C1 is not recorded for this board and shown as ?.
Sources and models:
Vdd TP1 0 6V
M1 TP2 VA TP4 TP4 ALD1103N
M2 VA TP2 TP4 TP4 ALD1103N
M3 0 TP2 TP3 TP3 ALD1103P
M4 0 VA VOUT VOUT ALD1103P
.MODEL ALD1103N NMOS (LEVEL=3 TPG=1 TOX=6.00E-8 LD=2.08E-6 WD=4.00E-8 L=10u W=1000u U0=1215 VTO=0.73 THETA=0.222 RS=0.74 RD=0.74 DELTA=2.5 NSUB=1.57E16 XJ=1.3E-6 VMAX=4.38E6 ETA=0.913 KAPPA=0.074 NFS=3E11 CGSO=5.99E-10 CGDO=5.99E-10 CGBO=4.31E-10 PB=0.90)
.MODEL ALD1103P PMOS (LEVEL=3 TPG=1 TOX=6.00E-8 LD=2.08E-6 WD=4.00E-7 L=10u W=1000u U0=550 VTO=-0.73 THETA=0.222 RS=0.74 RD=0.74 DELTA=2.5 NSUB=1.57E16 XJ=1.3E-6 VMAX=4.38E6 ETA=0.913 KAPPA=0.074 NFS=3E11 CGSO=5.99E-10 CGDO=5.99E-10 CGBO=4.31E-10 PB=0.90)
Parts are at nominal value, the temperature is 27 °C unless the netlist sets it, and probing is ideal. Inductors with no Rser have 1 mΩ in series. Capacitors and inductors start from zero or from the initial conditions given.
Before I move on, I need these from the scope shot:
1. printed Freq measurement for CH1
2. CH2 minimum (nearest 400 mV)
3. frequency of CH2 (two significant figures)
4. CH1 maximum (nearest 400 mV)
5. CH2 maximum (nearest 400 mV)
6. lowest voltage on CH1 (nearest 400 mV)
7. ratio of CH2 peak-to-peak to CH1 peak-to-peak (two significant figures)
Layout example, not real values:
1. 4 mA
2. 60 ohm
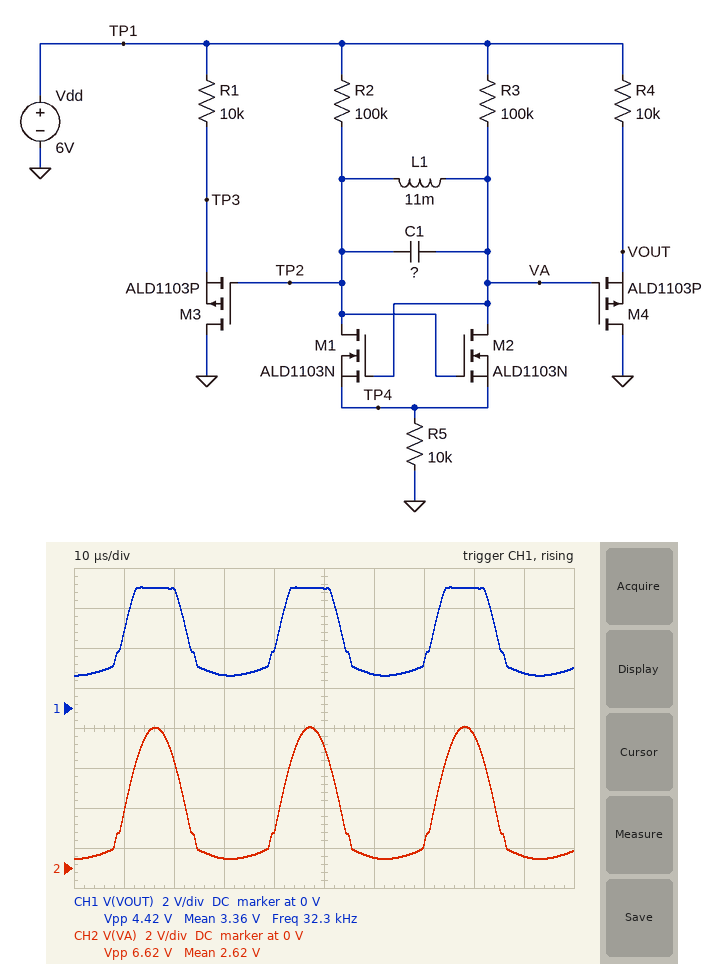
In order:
1. 32.3 kHz
2. 400 mV
3. 32 kHz
4. 6.0 V
5. 7.2 V
6. 1.6 V
7. 1.5
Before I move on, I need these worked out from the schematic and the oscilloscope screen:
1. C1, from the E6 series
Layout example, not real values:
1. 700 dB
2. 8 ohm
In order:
1. 2.2 nF
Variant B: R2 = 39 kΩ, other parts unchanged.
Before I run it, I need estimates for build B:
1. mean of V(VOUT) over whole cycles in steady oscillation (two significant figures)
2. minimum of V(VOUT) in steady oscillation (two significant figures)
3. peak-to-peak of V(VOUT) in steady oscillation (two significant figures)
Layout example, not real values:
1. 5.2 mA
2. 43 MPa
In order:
1. 3.7 V
2. 1.5 V
3. 4.5 V
